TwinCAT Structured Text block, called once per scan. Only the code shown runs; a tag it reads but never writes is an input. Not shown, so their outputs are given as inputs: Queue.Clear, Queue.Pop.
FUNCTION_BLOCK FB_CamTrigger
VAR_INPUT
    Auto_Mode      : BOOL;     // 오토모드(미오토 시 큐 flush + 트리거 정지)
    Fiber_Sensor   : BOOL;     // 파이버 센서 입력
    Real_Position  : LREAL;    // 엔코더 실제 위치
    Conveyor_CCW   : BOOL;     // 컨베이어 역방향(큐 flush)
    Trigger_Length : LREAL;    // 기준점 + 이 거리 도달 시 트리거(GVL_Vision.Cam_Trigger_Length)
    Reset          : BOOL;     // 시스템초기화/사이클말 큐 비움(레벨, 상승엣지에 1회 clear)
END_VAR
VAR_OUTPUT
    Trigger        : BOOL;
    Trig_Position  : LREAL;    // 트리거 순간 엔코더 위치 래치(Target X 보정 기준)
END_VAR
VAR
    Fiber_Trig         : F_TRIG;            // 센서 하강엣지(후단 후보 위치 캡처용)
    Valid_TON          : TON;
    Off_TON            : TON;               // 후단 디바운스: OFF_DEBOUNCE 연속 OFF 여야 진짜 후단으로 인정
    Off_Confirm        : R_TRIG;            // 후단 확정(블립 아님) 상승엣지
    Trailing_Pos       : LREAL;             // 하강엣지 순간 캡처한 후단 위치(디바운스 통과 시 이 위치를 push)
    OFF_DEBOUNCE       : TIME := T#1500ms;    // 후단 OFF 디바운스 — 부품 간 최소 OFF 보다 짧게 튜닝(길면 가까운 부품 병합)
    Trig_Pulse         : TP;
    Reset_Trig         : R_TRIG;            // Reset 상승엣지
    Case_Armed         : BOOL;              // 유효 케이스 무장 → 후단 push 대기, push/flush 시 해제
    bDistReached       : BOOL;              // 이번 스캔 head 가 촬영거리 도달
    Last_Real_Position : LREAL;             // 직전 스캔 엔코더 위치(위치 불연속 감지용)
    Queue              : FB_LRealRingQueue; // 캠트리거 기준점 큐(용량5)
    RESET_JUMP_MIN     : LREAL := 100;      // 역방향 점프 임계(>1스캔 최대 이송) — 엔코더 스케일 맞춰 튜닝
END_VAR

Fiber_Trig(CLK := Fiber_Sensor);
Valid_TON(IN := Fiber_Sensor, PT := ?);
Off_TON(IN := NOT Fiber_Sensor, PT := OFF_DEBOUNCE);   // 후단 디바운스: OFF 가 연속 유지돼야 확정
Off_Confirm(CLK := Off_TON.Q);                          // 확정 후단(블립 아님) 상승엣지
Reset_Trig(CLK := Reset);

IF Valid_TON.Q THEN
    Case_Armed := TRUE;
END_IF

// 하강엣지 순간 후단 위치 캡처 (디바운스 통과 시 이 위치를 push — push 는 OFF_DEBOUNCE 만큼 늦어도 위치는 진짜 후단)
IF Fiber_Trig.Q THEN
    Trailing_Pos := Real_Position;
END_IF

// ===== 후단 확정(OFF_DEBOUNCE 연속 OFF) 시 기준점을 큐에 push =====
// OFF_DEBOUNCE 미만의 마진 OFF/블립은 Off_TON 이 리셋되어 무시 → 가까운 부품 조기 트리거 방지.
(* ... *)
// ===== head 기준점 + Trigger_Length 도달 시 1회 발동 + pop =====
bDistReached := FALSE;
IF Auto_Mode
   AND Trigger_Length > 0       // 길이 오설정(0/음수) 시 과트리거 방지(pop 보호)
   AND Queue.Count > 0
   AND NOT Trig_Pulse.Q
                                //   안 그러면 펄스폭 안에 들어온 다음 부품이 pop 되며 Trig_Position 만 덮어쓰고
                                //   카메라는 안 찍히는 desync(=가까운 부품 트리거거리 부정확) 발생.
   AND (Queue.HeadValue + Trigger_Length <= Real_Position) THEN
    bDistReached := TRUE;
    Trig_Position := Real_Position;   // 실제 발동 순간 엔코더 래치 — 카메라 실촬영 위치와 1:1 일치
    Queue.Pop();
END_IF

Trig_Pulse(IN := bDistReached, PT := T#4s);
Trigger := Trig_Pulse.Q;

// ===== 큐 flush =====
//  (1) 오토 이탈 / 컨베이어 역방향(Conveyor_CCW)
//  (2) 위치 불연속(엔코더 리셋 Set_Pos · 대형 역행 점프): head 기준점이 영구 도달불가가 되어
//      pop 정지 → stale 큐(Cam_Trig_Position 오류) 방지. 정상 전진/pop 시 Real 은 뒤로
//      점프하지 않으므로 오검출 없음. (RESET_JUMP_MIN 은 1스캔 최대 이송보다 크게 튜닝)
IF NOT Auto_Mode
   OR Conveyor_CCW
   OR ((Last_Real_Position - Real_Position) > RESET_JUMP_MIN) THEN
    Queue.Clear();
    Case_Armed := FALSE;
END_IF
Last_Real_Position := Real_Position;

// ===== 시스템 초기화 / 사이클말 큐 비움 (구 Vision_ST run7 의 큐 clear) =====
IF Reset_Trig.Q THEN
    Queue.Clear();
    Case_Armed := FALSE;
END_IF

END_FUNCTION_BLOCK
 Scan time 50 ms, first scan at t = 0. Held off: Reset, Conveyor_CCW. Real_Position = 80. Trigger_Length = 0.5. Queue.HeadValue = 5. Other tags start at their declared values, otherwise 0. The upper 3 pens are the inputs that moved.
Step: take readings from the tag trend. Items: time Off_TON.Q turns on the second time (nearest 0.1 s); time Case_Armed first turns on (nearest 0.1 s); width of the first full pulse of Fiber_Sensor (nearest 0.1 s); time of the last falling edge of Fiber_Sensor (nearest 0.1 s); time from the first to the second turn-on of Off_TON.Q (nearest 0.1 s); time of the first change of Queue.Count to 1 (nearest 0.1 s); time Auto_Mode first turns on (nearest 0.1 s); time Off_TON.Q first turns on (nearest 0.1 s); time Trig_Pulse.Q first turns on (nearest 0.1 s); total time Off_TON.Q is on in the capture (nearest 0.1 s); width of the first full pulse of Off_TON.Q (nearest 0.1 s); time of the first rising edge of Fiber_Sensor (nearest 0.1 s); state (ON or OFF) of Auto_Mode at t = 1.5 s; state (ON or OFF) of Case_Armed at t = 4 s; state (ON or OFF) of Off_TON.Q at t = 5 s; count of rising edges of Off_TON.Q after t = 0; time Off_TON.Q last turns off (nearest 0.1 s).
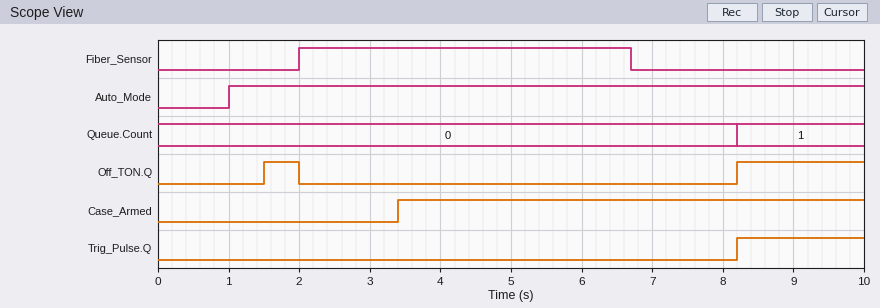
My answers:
8.2 s
3.4 s
4.7 s
6.7 s
6.7 s
8.2 s
1.0 s
1.5 s
8.2 s
2.3 s
0.5 s
2.0 s
ON
ON
OFF
2
2.0 s
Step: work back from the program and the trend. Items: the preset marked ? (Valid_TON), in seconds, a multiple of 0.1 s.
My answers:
1.4 s
